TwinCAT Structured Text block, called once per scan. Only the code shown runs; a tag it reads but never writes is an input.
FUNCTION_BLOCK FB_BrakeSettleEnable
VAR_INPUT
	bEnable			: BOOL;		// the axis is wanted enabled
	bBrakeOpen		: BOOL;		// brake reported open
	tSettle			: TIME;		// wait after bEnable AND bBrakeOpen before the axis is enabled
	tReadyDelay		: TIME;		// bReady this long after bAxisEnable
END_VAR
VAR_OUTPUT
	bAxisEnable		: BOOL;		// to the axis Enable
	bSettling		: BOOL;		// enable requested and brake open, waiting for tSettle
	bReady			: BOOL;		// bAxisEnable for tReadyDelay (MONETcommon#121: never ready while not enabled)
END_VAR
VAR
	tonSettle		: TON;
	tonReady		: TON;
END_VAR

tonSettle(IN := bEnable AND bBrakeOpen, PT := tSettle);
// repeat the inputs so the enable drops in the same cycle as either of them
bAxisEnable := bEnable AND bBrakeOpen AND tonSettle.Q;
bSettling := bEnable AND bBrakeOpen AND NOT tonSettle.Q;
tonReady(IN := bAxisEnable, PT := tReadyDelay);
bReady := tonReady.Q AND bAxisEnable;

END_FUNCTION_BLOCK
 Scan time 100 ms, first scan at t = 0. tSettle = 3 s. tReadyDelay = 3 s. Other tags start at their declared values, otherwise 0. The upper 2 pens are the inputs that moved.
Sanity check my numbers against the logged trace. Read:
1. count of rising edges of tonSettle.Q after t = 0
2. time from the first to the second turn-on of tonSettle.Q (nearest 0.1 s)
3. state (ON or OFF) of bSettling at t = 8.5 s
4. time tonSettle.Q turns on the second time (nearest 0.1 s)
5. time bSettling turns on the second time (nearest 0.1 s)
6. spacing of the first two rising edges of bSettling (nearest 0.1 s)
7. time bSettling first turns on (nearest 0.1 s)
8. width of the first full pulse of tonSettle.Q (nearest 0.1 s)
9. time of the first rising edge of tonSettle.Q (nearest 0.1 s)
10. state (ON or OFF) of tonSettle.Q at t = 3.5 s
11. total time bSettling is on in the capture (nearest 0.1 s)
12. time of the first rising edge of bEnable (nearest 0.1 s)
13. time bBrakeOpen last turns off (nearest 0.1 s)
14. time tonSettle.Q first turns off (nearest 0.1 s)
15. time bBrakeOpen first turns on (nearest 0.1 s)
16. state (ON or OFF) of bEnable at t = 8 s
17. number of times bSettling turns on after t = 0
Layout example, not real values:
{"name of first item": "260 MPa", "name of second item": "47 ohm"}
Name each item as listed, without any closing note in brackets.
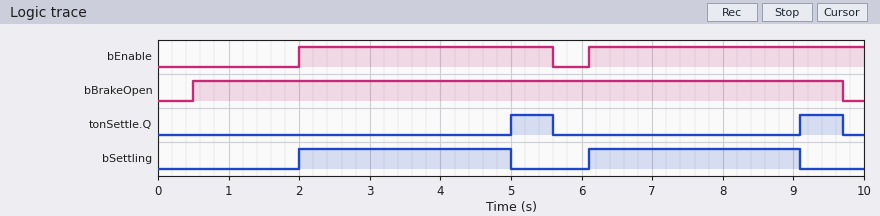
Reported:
{"count of rising edges of tonSettle.Q after t = 0": "2", "time from the first to the second turn-on of tonSettle.Q": "4.1 s", "state (ON or OFF) of bSettling at t = 8.5 s": "ON", "time tonSettle.Q turns on the second time": "9.1 s", "time bSettling turns on the second time": "6.1 s", "spacing of the first two rising edges of bSettling": "4.1 s", "time bSettling first turns on": "2.0 s", "width of the first full pulse of tonSettle.Q": "0.6 s", "time of the first rising edge of tonSettle.Q": "5.0 s", "state (ON or OFF) of tonSettle.Q at t = 3.5 s": "OFF", "total time bSettling is on in the capture": "6.0 s", "time of the first rising edge of bEnable": "2.0 s", "time bBrakeOpen last turns off": "9.7 s", "time tonSettle.Q first turns off": "5.6 s", "time bBrakeOpen first turns on": "0.5 s", "state (ON or OFF) of bEnable at t = 8 s": "ON", "number of times bSettling turns on after t = 0": "2"}
